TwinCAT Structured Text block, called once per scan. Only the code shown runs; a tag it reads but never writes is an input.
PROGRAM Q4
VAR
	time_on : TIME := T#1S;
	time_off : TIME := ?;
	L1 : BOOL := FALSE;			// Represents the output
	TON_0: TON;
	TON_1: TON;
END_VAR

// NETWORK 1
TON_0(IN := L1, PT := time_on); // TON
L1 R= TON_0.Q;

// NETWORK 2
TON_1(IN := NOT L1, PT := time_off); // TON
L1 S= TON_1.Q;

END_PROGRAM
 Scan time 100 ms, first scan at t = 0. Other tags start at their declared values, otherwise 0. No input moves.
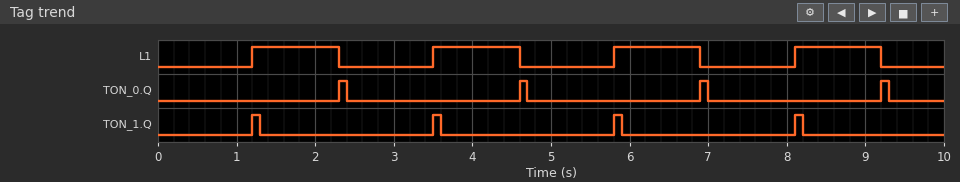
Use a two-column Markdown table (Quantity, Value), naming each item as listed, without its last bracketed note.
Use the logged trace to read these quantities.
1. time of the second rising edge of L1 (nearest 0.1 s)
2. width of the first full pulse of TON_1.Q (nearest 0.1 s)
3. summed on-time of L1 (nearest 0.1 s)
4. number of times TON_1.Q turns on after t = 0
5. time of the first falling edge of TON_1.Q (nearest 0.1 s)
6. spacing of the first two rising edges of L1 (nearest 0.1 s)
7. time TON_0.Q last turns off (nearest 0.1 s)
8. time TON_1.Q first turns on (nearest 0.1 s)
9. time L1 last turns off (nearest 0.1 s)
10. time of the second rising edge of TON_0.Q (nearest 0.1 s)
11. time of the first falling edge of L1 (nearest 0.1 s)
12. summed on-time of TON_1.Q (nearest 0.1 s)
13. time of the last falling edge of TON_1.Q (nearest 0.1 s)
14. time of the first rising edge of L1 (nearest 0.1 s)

| Quantity | Value |
|---|---|
| time of the second rising edge of L1 | 3.5 s |
| width of the first full pulse of TON_1.Q | 0.1 s |
| summed on-time of L1 | 4.4 s |
| number of times TON_1.Q turns on after t = 0 | 4 |
| time of the first falling edge of TON_1.Q | 1.3 s |
| spacing of the first two rising edges of L1 | 2.3 s |
| time TON_0.Q last turns off | 9.3 s |
| time TON_1.Q first turns on | 1.2 s |
| time L1 last turns off | 9.2 s |
| time of the second rising edge of TON_0.Q | 4.6 s |
| time of the first falling edge of L1 | 2.3 s |
| summed on-time of TON_1.Q | 0.4 s |
| time of the last falling edge of TON_1.Q | 8.2 s |
| time of the first rising edge of L1 | 1.2 s |
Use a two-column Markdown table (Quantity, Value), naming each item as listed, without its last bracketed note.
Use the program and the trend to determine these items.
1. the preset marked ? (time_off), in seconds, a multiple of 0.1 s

| Quantity | Value |
|---|---|
| the preset marked ? (time_off), in seconds, a multiple of 0.1 s | 1.2 s |
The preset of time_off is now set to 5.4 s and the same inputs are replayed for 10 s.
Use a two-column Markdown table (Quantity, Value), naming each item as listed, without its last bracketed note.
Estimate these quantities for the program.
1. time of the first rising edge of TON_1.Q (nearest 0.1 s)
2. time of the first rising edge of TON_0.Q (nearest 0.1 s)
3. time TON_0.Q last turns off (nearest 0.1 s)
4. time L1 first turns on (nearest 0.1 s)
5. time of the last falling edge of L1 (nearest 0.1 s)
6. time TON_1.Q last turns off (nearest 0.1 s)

| Quantity | Value |
|---|---|
| time of the first rising edge of TON_1.Q | 5.4 s |
| time of the first rising edge of TON_0.Q | 6.5 s |
| time TON_0.Q last turns off | 6.6 s |
| time L1 first turns on | 5.4 s |
| time of the last falling edge of L1 | 6.5 s |
| time TON_1.Q last turns off | 5.5 s |
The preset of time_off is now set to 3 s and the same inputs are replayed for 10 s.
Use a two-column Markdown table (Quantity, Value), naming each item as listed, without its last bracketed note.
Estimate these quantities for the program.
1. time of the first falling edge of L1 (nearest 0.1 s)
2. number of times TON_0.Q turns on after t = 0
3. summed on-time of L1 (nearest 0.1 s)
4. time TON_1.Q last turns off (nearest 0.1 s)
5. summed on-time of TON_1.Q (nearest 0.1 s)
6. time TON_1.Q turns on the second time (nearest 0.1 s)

| Quantity | Value |
|---|---|
| time of the first falling edge of L1 | 4.1 s |
| number of times TON_0.Q turns on after t = 0 | 2 |
| summed on-time of L1 | 2.2 s |
| time TON_1.Q last turns off | 7.2 s |
| summed on-time of TON_1.Q | 0.2 s |
| time TON_1.Q turns on the second time | 7.1 s |
